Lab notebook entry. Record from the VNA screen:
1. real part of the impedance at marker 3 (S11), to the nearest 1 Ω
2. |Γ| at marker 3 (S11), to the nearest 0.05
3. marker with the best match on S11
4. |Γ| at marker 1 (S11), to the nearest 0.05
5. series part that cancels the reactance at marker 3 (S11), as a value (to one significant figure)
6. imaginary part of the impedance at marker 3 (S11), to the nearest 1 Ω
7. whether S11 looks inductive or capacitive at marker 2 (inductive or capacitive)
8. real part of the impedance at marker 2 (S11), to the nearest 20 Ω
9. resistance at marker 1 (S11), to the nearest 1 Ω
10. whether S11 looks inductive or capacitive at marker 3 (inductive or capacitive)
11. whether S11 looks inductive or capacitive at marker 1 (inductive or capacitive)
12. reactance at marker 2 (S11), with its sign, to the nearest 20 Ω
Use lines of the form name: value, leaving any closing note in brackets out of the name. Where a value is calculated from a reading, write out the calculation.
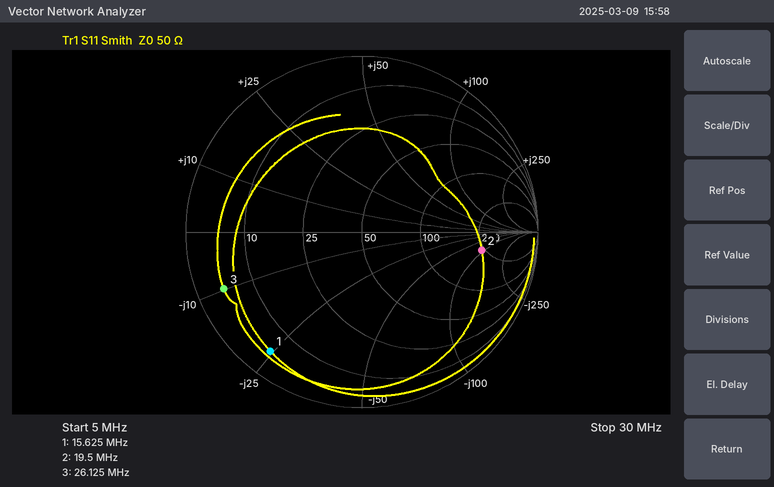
real part of the impedance at marker 3 (S11), to the nearest 1 Ω: 4 Ω
|Γ| at marker 3 (S11), to the nearest 0.05: 0.85
marker with the best match on S11: marker 2
|Γ| at marker 1 (S11), to the nearest 0.05: 0.85
series part that cancels the reactance at marker 3 (S11), as a value: L = 10 Ω/(2π × 26.125 MHz) ≈ 60.9 nH, so 60 nH to one significant figure
imaginary part of the impedance at marker 3 (S11), to the nearest 1 Ω: -10 Ω
whether S11 looks inductive or capacitive at marker 2: capacitive
real part of the impedance at marker 2 (S11), to the nearest 20 Ω: 240 Ω
resistance at marker 1 (S11), to the nearest 1 Ω: 5 Ω
whether S11 looks inductive or capacitive at marker 3: capacitive
whether S11 looks inductive or capacitive at marker 1: capacitive
reactance at marker 2 (S11), with its sign, to the nearest 20 Ω: -100 Ω
